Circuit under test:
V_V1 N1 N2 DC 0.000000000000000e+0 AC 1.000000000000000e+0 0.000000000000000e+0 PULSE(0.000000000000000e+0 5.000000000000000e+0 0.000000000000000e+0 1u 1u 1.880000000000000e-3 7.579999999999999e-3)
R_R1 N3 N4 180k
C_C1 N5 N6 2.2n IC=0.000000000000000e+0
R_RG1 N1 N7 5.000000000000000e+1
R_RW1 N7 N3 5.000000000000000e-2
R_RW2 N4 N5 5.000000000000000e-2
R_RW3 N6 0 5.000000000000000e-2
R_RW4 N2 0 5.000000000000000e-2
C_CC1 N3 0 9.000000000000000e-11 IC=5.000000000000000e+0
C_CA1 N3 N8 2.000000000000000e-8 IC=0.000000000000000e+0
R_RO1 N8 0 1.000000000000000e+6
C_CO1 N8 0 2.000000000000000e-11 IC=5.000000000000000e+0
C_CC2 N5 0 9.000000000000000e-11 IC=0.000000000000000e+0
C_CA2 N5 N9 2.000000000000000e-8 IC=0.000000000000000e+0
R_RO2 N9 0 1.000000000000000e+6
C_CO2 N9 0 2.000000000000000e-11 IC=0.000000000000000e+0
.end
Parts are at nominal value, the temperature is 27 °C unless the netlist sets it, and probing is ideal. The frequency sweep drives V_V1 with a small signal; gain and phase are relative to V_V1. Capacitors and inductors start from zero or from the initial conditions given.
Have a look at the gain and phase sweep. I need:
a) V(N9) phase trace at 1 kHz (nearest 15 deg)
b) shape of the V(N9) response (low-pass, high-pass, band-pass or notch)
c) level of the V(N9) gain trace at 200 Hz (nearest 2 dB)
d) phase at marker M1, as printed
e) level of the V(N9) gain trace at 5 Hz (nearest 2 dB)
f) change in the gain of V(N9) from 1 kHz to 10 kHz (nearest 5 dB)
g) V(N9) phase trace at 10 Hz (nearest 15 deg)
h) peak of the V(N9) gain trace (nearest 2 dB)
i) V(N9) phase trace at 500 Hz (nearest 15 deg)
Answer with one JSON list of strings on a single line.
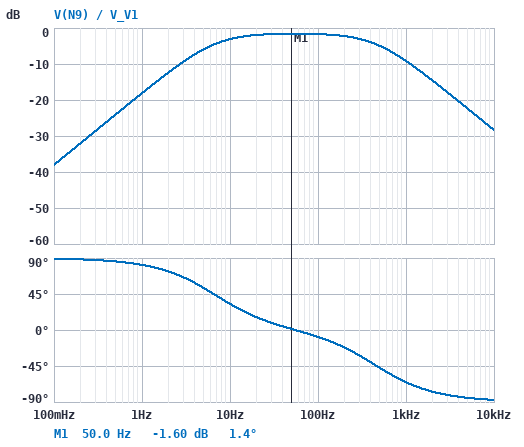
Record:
["-60 deg", "band-pass", "-2 dB", "1.4 deg", "-6 dB", "-20 dB", "30 deg", "-2 dB", "-45 deg"]
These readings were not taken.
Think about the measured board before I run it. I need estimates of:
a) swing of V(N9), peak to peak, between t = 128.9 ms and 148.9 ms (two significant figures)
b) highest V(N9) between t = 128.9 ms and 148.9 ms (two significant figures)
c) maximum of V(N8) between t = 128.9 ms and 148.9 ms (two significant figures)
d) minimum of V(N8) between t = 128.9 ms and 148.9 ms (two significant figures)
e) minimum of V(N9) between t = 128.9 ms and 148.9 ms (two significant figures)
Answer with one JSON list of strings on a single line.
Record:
["4.2 V", "3.1 V", "3.9 V", "-1.4 V", "-1.1 V"]
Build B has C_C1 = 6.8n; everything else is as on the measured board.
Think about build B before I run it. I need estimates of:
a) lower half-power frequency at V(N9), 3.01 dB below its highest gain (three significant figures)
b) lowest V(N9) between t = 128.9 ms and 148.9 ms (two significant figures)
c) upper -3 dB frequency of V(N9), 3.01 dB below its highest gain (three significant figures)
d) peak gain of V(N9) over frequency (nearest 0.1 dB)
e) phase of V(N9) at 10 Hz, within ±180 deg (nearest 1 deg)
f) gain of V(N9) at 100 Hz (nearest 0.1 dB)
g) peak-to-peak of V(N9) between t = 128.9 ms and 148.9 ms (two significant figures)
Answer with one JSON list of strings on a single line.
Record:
["6.16 Hz", "-960 mV", "165 Hz", "-1.9 dB", "30 deg", "-3.1 dB", "3.4 V"]
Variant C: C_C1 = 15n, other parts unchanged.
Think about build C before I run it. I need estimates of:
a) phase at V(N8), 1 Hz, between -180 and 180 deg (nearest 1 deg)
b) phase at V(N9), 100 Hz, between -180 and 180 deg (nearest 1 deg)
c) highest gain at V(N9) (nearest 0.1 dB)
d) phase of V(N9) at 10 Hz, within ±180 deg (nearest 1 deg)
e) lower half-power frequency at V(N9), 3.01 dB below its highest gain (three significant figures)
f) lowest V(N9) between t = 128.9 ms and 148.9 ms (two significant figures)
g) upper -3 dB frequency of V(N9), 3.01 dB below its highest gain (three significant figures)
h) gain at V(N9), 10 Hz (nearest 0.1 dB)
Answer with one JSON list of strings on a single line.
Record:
["83 deg", "-51 deg", "-2.4 dB", "25 deg", "5.63 Hz", "-790 mV", "82.6 Hz", "-3.3 dB"]
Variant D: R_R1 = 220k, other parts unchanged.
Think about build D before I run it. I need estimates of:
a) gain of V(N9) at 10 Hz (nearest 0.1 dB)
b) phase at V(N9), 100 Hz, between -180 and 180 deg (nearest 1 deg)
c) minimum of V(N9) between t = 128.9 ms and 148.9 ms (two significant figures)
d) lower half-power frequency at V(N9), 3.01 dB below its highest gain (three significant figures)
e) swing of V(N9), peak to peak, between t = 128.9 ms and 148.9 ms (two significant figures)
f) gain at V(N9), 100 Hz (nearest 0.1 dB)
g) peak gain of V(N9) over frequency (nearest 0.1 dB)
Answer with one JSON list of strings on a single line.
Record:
["-3.3 dB", "-11 deg", "-1.0 V", "6.28 Hz", "4.0 V", "-2.1 dB", "-1.9 dB"]
